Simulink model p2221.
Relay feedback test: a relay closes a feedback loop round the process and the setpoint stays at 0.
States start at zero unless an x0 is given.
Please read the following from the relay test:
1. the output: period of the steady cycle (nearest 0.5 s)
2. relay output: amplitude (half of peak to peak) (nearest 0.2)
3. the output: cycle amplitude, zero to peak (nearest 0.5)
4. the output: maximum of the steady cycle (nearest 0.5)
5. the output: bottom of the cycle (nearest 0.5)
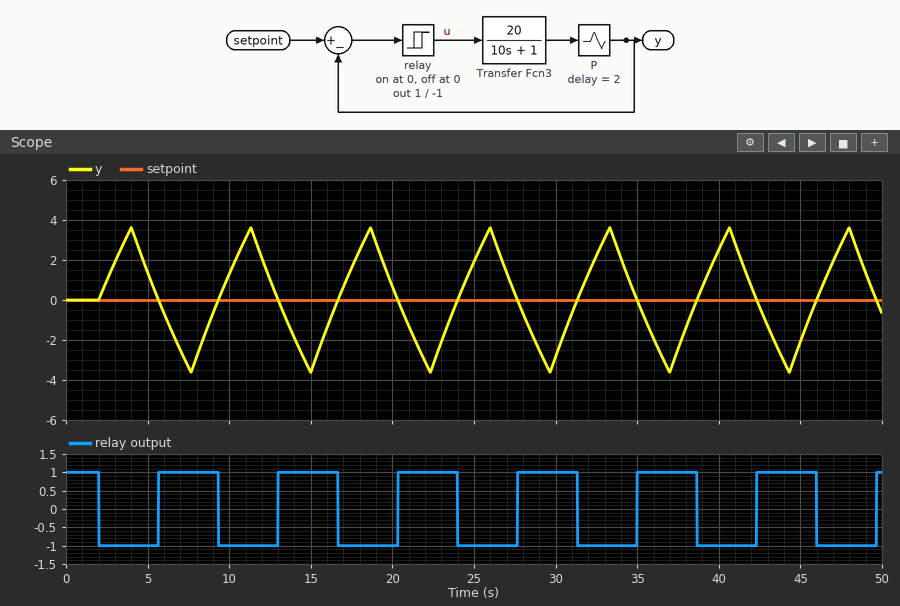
7.5 s
1.0
3.5
3.5
-3.5
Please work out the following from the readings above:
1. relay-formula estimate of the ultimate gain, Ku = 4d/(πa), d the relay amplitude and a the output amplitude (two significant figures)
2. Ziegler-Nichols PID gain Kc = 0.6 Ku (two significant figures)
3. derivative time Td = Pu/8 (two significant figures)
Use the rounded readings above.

0.36
0.22
0.94 s
